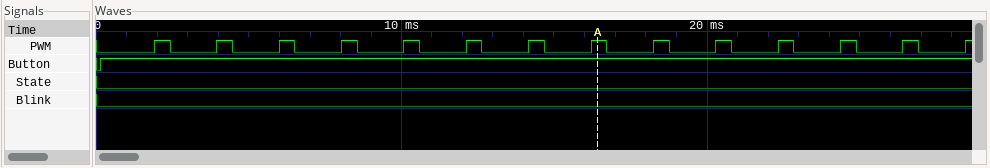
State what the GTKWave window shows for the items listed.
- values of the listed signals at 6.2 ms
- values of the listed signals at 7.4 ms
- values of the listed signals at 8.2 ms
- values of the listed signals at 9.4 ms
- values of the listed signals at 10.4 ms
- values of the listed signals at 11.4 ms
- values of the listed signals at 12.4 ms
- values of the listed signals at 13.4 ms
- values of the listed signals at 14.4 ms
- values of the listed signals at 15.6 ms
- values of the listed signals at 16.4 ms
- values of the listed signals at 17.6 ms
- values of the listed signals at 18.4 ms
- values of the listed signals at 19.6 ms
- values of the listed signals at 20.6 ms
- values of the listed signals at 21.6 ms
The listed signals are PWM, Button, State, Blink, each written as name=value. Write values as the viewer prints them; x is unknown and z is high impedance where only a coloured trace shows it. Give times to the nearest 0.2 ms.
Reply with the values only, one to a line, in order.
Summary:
PWM=1, Button=1, State=0, Blink=0
PWM=0, Button=1, State=0, Blink=0
PWM=1, Button=1, State=0, Blink=0
PWM=0, Button=1, State=0, Blink=0
PWM=1, Button=1, State=0, Blink=0
PWM=0, Button=1, State=0, Blink=0
PWM=1, Button=1, State=0, Blink=0
PWM=0, Button=1, State=0, Blink=0
PWM=1, Button=1, State=0, Blink=0
PWM=0, Button=1, State=0, Blink=0
PWM=1, Button=1, State=0, Blink=0
PWM=0, Button=1, State=0, Blink=0
PWM=1, Button=1, State=0, Blink=0
PWM=0, Button=1, State=0, Blink=0
PWM=1, Button=1, State=0, Blink=0
PWM=0, Button=1, State=0, Blink=0
